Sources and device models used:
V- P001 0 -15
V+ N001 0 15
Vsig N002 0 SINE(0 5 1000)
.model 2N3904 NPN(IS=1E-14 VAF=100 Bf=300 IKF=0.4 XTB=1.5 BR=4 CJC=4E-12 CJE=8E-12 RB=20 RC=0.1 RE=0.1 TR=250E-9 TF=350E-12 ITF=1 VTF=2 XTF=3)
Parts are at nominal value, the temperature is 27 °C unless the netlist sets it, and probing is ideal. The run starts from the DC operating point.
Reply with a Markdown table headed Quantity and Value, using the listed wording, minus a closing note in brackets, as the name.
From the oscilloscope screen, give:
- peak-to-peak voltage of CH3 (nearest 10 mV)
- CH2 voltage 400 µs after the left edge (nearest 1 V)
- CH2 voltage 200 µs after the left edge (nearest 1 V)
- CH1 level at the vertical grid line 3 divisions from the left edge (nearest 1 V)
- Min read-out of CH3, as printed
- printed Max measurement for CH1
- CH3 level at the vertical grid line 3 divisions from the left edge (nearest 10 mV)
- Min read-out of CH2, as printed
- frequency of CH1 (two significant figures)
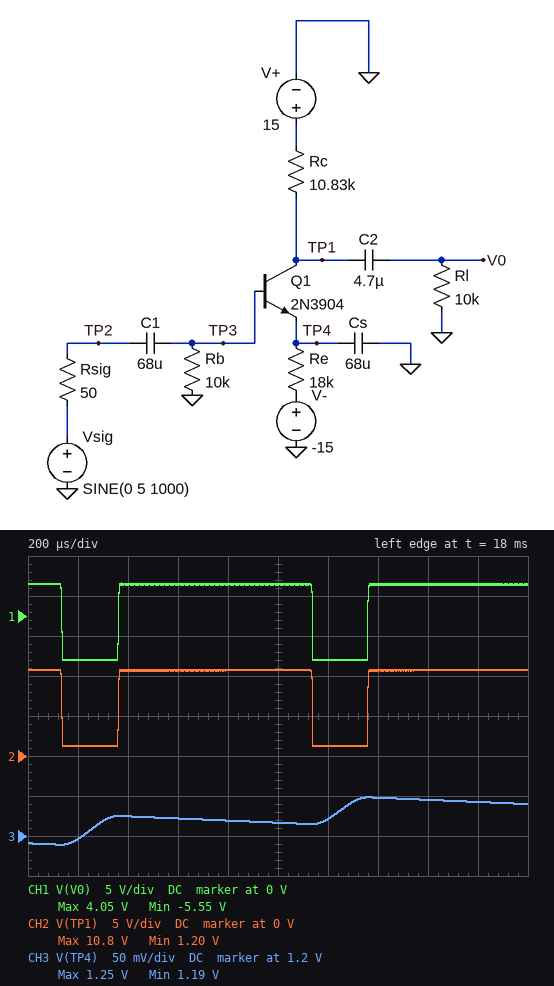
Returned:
| Quantity | Value |
|---|---|
| peak-to-peak voltage of CH3 | 60 mV |
| CH2 voltage 400 µs after the left edge | 11 V |
| CH2 voltage 200 µs after the left edge | 1 V |
| CH1 level at the vertical grid line 3 divisions from the left edge | 4 V |
| Min read-out of CH3, as printed | 1.19 V |
| printed Max measurement for CH1 | 4.05 V |
| CH3 level at the vertical grid line 3 divisions from the left edge | 1.22 V |
| Min read-out of CH2, as printed | 1.20 V |
| frequency of CH1 | 1.0 kHz |
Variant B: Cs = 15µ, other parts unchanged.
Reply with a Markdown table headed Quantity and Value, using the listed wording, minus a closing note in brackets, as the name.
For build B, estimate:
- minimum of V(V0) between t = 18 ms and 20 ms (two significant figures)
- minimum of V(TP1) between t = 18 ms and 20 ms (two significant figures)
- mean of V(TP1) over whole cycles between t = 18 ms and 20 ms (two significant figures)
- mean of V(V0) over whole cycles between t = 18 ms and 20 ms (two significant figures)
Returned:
| Quantity | Value |
|---|---|
| minimum of V(V0) between t = 18 ms and 20 ms | -4.4 V |
| minimum of V(TP1) between t = 18 ms and 20 ms | 2.8 V |
| mean of V(TP1) over whole cycles between t = 18 ms and 20 ms | 9.6 V |
| mean of V(V0) over whole cycles between t = 18 ms and 20 ms | 2.4 V |
